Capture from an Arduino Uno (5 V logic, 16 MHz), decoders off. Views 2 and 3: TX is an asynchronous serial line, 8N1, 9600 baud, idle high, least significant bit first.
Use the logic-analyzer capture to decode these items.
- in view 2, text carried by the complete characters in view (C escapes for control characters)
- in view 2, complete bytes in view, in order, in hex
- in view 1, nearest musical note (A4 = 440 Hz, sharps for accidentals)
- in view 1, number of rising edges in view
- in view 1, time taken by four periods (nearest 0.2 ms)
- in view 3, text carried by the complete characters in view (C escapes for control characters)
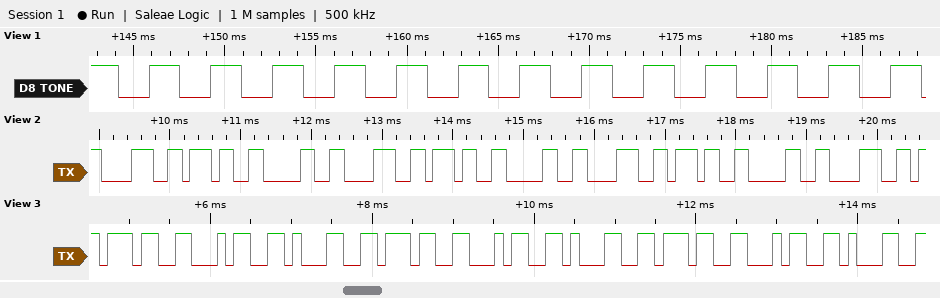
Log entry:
"8708708708"
38 37 30 38 37 30 38 37 30 38
D4
13
13.6 ms
"741741741"
